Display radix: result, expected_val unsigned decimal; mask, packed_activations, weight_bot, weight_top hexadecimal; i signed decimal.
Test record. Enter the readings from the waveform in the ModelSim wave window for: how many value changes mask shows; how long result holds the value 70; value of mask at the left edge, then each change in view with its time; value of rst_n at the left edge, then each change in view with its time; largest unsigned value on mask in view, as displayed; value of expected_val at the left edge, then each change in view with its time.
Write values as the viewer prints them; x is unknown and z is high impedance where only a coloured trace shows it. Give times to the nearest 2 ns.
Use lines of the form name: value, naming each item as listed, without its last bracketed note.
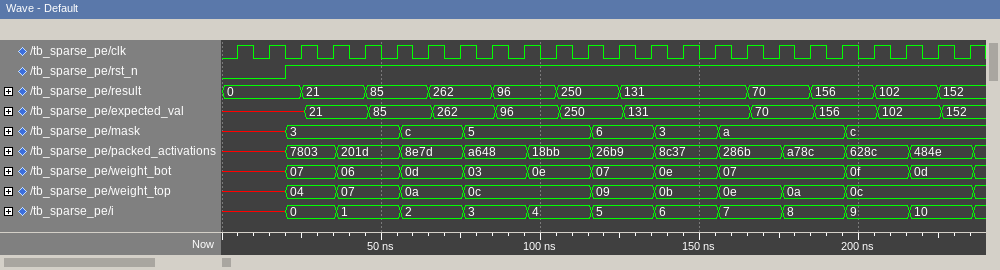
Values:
how many value changes mask shows: 7
how long result holds the value 70: 20 ns
value of mask at the left edge, then each change in view with its time: x, 3 at 20 ns, c at 56 ns, 5 at 76 ns, 6 at 116 ns, 3 at 136 ns, a at 156 ns, c at 196 ns
value of rst_n at the left edge, then each change in view with its time: 0, 1 at 20 ns
largest unsigned value on mask in view, as displayed: c
value of expected_val at the left edge, then each change in view with its time: x, 21 at 26 ns, 85 at 46 ns, 262 at 66 ns, 96 at 86 ns, 250 at 106 ns, 131 at 126 ns, 70 at 166 ns, 156 at 186 ns, 102 at 206 ns, 152 at 226 ns
